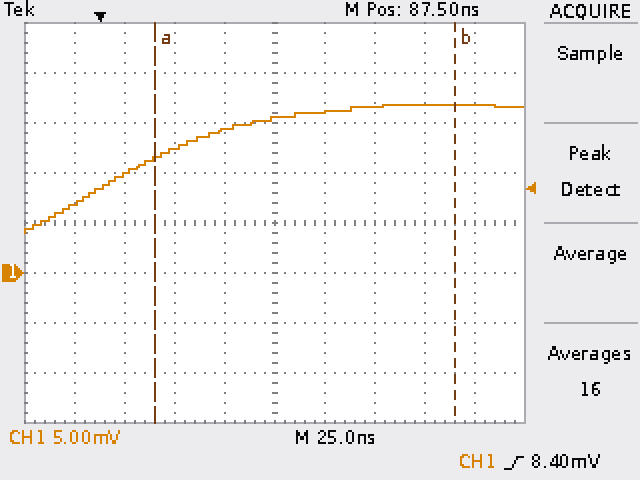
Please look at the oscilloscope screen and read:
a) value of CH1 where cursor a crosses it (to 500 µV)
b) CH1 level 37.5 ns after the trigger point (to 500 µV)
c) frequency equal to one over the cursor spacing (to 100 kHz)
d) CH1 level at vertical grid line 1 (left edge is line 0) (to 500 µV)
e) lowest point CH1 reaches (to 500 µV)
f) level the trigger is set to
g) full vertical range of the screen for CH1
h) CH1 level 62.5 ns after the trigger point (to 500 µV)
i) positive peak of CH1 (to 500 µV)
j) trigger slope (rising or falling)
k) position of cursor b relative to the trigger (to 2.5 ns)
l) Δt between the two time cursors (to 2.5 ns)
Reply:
11.5 mV
12.5 mV
6.7 MHz
7.0 mV
4.0 mV
8.40 mV
40 mV
14.5 mV
17.0 mV
rising
+177.5 ns
150.0 ns
